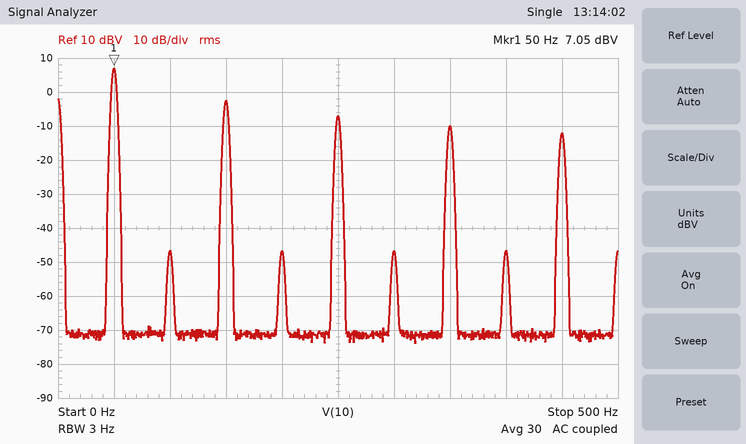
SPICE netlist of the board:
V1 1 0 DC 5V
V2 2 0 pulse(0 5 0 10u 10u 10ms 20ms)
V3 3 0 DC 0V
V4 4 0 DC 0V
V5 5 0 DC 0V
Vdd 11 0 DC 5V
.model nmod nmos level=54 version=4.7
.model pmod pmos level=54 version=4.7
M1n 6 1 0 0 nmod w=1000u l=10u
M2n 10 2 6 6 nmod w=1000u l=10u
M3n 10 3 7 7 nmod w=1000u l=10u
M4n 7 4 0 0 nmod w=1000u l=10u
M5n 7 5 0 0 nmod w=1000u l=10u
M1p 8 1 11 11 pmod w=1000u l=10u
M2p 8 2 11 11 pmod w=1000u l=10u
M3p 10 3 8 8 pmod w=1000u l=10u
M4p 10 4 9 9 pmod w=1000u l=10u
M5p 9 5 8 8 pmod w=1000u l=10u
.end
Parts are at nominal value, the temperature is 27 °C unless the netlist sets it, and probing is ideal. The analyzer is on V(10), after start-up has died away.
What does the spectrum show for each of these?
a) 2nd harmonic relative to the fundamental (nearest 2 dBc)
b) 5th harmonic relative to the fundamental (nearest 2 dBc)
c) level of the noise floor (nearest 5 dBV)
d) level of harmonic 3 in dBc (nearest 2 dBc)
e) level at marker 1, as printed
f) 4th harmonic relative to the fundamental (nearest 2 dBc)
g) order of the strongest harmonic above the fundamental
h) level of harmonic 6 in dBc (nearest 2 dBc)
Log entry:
-54 dBc
-14 dBc
-70 dBV
-10 dBc
7.05 dBV
-54 dBc
3
-54 dBc
